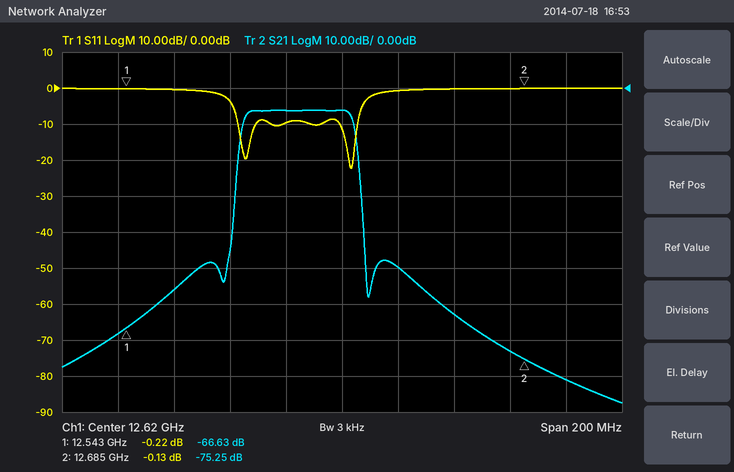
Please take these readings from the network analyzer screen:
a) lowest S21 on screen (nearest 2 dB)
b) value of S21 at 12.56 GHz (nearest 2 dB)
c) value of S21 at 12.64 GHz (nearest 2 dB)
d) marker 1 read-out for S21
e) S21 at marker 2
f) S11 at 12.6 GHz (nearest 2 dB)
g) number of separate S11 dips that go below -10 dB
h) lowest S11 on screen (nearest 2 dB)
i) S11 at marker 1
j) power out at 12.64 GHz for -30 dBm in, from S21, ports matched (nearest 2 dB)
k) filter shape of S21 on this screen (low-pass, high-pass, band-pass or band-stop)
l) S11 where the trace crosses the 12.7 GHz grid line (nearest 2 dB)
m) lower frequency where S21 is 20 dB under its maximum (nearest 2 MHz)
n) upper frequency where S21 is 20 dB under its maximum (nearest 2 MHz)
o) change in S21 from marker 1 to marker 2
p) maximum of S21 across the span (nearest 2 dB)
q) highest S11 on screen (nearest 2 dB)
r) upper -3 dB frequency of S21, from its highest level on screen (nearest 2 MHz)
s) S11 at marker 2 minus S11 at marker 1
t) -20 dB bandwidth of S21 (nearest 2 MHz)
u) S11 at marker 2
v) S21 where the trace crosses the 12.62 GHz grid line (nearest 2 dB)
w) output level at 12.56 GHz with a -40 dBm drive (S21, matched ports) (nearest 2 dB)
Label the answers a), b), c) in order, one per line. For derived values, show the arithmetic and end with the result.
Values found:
a) -88 dB
b) -56 dB
c) -50 dB
d) -66.63 dB
e) -75.25 dB
f) -10 dB
g) 2
h) -22 dB
i) -0.22 dB
j) -30 dBm + (-50 dB) = -80 dBm
k) band-pass
l) 0 dB
m) 12.582 GHz
n) 12.626 GHz
o) -75.25 − (-66.63) = -8.62 dB
p) -6 dB
q) 0 dB
r) 12.624 GHz
s) -0.13 − (-0.22) = 0.09 dB
t) 12.626 GHz − 12.582 GHz = 44 MHz
u) -0.13 dB
v) -6 dB
w) -40 dBm + (-56 dB) = -96 dBm
